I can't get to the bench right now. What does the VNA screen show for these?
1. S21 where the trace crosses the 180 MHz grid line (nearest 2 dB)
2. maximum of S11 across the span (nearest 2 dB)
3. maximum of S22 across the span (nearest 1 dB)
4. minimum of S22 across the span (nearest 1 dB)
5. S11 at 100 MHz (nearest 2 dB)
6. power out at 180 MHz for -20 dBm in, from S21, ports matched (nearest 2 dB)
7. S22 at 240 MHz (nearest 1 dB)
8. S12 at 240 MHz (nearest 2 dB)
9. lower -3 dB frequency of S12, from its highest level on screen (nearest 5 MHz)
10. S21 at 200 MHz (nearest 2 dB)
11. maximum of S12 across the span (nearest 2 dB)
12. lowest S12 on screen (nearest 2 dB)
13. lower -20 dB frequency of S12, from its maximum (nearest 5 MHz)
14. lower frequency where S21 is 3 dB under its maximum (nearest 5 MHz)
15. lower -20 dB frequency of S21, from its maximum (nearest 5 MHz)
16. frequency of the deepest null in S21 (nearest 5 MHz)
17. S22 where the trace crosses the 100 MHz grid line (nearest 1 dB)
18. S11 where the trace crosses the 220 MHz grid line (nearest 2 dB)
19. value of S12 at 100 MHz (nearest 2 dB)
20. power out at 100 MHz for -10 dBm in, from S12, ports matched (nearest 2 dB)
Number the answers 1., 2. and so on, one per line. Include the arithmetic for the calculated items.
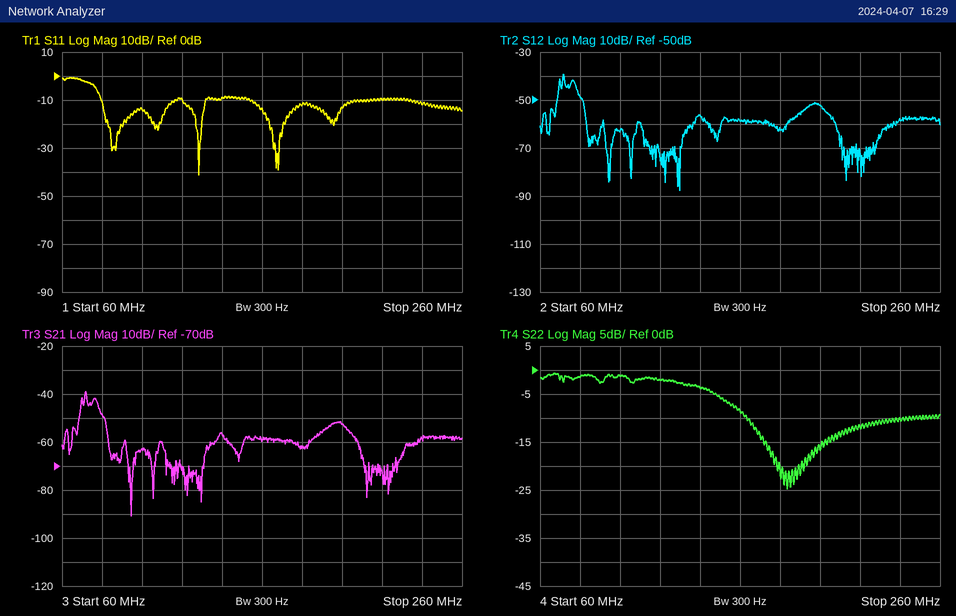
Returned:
1. -62 dB
2. 0 dB
3. -1 dB
4. -25 dB
5. -14 dB
6. -20 dBm + (-62 dB) = -82 dBm
7. -10 dB
8. -58 dB
9. 70 MHz
10. -52 dB
11. -40 dB
12. -88 dB
13. 65 MHz
14. 70 MHz
15. 65 MHz
16. 95 MHz
17. -1 dB
18. -10 dB
19. -62 dB
20. -10 dBm + (-62 dB) = -72 dBm
